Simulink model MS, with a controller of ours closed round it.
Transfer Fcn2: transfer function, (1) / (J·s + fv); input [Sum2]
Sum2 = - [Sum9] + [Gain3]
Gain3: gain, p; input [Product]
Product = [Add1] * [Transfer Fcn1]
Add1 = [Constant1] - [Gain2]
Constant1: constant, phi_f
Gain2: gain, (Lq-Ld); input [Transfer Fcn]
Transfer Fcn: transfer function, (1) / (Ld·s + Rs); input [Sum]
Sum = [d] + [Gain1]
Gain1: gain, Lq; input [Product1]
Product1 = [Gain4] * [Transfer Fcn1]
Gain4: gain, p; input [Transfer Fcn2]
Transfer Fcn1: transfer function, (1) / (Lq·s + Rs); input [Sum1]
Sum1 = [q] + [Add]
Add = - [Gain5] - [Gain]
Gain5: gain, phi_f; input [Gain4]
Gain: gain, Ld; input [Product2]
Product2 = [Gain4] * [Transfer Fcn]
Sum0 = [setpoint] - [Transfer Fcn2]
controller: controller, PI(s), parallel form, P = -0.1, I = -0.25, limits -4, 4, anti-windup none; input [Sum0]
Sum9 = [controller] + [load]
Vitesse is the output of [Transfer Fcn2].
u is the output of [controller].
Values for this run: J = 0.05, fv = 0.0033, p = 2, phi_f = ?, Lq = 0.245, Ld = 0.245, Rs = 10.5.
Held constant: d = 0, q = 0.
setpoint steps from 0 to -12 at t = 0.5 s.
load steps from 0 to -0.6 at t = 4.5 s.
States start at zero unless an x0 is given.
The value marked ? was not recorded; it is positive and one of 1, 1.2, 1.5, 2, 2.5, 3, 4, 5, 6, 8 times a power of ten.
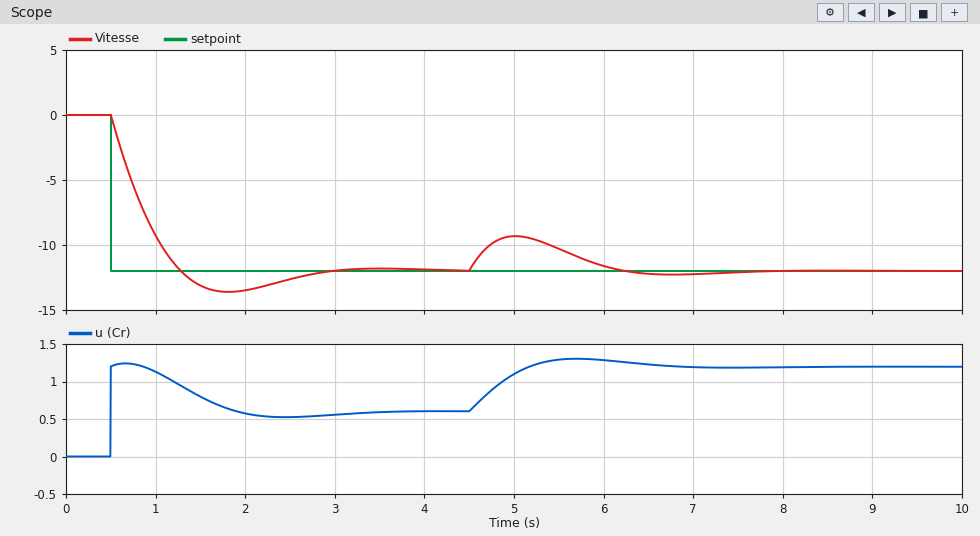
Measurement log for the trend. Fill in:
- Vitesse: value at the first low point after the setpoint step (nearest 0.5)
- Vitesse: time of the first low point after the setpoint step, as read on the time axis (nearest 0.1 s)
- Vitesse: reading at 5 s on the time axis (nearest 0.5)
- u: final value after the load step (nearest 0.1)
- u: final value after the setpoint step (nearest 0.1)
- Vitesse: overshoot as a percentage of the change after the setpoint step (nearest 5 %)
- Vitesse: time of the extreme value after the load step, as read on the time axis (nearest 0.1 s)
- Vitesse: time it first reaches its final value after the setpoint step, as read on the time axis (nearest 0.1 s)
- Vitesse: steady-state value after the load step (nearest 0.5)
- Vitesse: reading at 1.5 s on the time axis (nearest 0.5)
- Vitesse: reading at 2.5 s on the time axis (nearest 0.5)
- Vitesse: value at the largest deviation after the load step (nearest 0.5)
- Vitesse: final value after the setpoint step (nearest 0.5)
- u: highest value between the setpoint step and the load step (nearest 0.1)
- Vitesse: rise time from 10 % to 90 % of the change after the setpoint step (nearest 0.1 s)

-13.5
1.8 s
-9.5
1.2
0.6
15 %
5.0 s
1.3 s
-12.0
-13.0
-12.5
-9.5
-12.0
1.2
0.6 s
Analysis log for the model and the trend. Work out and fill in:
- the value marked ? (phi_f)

0.4
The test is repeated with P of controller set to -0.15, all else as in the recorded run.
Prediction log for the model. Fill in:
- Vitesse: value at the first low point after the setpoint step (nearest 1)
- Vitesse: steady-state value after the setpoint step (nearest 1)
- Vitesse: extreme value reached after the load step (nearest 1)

-13
-12
-10
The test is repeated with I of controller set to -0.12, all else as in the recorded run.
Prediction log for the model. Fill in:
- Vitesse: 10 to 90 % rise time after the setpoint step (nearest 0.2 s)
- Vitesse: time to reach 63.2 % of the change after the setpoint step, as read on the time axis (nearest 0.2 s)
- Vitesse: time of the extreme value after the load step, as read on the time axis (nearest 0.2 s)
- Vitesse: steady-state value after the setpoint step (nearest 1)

1.0 s
1.0 s
5.2 s
-12
